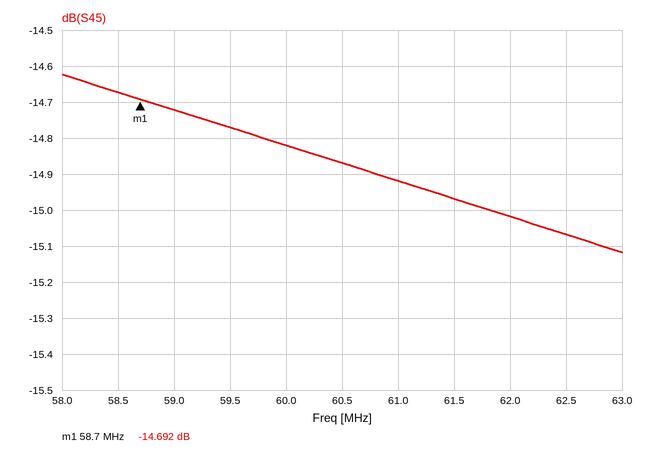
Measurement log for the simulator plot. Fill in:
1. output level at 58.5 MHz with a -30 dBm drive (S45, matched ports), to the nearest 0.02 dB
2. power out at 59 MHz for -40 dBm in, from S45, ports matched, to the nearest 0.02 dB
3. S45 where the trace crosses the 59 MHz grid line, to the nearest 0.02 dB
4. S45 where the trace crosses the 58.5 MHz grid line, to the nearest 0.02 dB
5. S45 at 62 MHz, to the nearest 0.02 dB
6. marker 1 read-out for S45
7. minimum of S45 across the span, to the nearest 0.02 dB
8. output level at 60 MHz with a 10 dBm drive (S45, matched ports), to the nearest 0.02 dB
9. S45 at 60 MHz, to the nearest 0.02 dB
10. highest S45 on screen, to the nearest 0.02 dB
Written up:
-44.68 dBm
-54.72 dBm
-14.72 dB
-14.68 dB
-15.02 dB
-14.692 dB
-15.12 dB
-4.82 dBm
-14.82 dB
-14.62 dB
